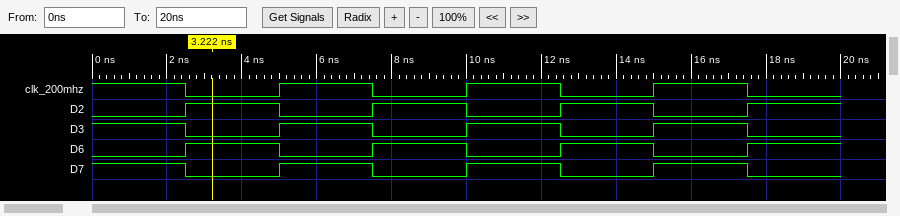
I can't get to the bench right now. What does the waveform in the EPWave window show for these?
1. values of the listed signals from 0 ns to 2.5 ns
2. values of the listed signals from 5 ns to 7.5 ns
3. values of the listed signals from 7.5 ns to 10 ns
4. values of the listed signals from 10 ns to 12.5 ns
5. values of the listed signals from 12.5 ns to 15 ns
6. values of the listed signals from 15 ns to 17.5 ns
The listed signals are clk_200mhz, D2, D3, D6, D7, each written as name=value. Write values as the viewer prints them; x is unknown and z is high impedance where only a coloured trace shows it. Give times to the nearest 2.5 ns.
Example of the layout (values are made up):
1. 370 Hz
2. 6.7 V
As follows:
1. clk_200mhz=1, D2=0, D3=1, D6=0, D7=1
2. clk_200mhz=1, D2=0, D3=1, D6=0, D7=1
3. clk_200mhz=0, D2=1, D3=0, D6=1, D7=0
4. clk_200mhz=1, D2=0, D3=1, D6=0, D7=1
5. clk_200mhz=0, D2=1, D3=0, D6=1, D7=0
6. clk_200mhz=1, D2=0, D3=1, D6=0, D7=1
